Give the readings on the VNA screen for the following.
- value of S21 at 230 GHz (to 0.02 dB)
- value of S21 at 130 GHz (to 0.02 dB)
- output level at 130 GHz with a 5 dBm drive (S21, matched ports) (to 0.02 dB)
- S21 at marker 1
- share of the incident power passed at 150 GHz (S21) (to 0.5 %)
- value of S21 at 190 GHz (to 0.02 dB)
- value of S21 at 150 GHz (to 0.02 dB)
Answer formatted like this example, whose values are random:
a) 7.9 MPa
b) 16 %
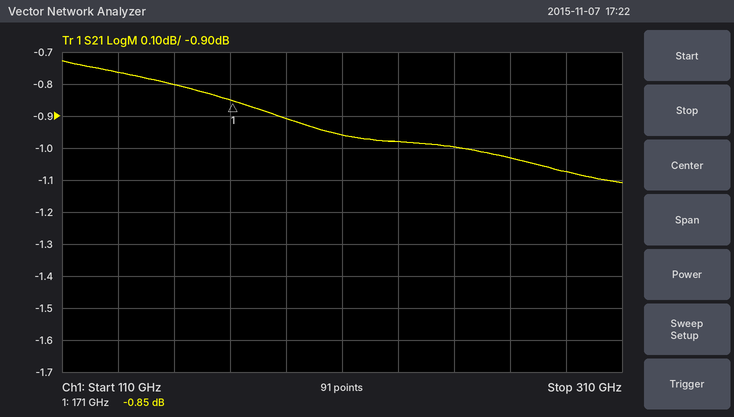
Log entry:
a) -0.98 dB
b) -0.76 dB
c) 4.24 dBm
d) -0.85 dB
e) 83.0 %
f) -0.90 dB
g) -0.80 dB
